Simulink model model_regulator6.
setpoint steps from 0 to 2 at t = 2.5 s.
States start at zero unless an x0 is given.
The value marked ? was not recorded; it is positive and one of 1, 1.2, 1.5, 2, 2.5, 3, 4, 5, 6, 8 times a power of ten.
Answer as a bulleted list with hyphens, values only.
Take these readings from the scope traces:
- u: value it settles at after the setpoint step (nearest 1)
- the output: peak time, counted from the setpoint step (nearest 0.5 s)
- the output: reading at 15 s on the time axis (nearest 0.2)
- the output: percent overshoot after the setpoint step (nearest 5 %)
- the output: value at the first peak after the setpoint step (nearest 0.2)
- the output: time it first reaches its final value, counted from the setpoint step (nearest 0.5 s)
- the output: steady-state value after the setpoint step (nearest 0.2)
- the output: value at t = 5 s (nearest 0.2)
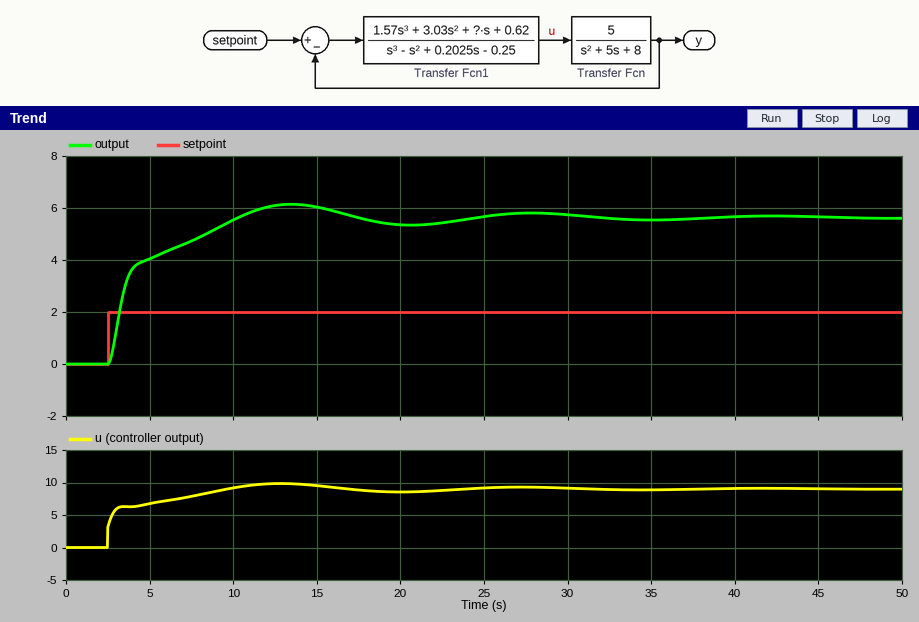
- 9
- 11.0 s
- 6.0
- 10 %
- 6.2
- 8.0 s
- 5.6
- 4.0
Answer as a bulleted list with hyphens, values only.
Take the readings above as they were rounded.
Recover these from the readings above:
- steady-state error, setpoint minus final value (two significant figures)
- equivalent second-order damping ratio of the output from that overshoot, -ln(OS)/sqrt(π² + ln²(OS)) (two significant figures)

- -3.6
- 0.59
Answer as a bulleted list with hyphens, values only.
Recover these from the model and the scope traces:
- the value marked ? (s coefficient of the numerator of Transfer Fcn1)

- 0.5
